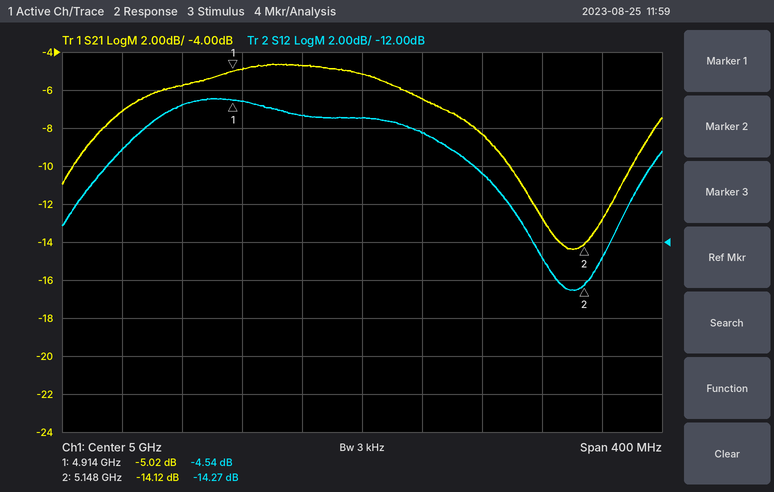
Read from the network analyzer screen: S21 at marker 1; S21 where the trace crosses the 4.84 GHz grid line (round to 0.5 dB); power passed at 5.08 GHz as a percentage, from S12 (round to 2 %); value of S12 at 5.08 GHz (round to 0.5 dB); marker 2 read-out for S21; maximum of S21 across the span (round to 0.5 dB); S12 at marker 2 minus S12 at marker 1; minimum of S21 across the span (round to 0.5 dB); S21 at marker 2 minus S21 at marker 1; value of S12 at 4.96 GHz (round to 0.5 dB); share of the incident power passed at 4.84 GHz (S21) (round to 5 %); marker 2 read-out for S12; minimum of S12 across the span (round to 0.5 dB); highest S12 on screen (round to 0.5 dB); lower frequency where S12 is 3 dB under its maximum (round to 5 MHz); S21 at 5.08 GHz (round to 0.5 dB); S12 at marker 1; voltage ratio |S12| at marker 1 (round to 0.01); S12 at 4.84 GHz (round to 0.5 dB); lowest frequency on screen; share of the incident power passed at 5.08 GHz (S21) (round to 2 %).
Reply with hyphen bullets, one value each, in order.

- -5.02 dB
- -7.0 dB
- 14 %
- -8.5 dB
- -14.12 dB
- -4.5 dB
- -9.73 dB
- -14.5 dB
- -9.10 dB
- -5.5 dB
- 20 %
- -14.27 dB
- -14.5 dB
- -4.5 dB
- 4.835 GHz
- -8.5 dB
- -4.54 dB
- 0.59
- -7.0 dB
- 4.8 GHz
- 14 %
